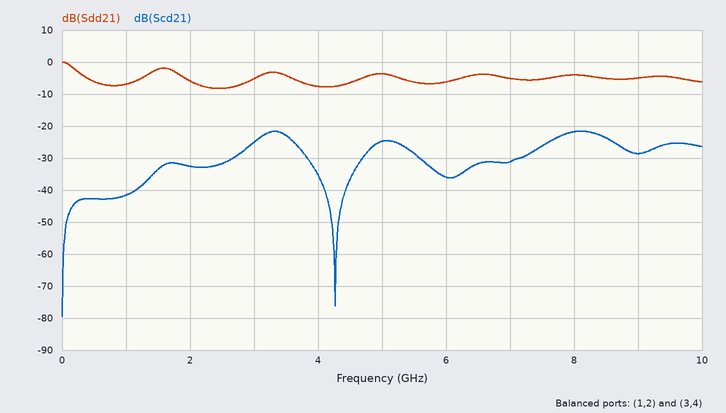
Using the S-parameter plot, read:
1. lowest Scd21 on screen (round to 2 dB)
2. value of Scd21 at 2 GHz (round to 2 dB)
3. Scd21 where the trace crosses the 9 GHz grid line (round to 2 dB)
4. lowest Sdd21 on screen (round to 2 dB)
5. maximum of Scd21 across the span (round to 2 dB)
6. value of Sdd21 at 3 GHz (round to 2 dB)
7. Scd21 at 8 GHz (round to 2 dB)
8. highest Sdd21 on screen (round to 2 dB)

-80 dB
-32 dB
-28 dB
-8 dB
-22 dB
-6 dB
-22 dB
0 dB
